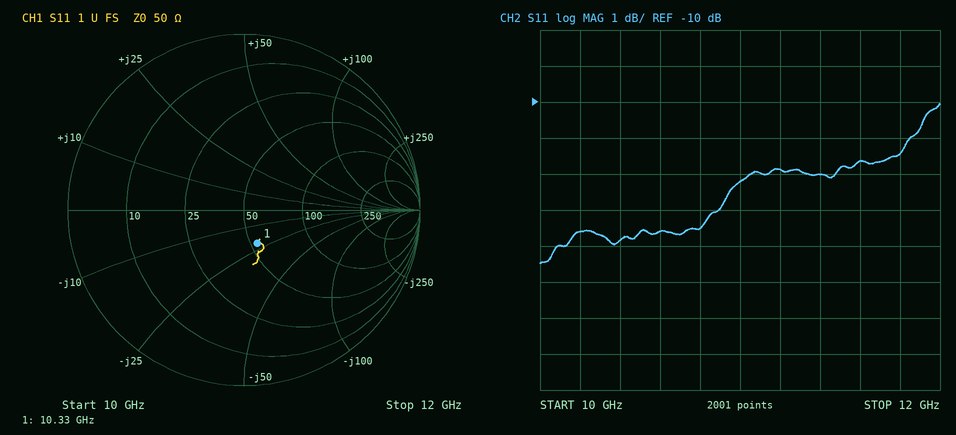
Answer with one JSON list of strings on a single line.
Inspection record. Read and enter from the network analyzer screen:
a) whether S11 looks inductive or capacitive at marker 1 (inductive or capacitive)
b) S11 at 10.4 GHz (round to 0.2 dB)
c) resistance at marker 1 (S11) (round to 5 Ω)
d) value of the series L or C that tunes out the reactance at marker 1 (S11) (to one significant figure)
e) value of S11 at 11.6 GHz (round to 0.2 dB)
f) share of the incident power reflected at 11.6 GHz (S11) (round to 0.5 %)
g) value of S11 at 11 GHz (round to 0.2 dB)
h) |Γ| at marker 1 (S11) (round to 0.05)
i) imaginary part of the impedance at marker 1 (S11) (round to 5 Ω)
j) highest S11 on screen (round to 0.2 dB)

["capacitive", "-13.8 dB", "55 Ω", "300 pH", "-11.6 dB", "7.0 %", "-12.2 dB", "0.20", "-20 Ω", "-10.0 dB"]
